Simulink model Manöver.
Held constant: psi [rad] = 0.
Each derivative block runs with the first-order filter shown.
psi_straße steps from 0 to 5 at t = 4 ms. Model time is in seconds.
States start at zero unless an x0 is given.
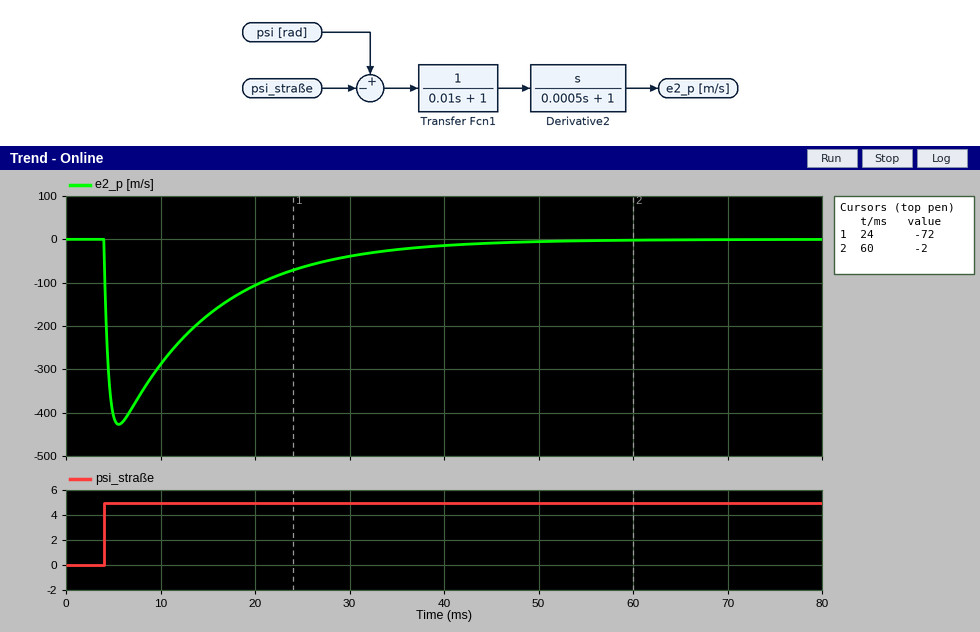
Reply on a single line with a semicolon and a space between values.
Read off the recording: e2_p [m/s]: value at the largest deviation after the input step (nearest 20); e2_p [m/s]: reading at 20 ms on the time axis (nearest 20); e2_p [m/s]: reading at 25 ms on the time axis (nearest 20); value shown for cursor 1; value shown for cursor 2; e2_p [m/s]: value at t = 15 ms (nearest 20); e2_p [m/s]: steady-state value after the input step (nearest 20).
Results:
-420; -100; -60; -72; -2; -180; 0
